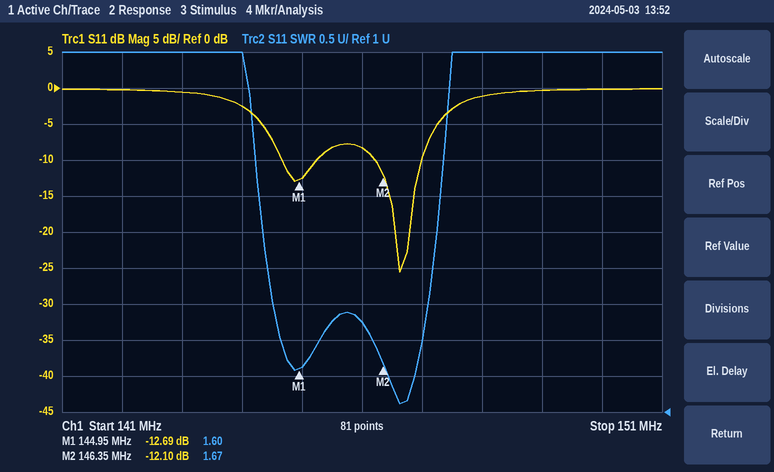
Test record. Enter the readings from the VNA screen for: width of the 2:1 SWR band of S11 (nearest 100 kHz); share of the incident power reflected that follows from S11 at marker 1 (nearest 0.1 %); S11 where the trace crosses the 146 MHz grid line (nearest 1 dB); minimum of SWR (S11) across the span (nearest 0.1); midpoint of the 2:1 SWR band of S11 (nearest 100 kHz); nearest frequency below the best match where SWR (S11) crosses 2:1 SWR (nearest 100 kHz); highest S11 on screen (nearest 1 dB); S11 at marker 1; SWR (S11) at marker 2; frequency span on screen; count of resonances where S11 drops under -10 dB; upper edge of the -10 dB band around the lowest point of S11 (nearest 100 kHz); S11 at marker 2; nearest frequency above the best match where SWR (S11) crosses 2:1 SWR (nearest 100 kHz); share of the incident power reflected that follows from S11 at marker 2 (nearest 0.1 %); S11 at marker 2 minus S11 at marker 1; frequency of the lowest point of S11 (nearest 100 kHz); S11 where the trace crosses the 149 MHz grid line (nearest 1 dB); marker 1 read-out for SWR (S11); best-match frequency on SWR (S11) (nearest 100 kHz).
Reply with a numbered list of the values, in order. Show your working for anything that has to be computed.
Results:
1. 147.0 MHz − 146.2 MHz = 800 kHz
2. 10^(-12.69/10) ≈ 5.4 %
3. -8 dB
4. 1.1
5. 146.6 MHz
6. 146.2 MHz
7. 0 dB
8. -12.69 dB
9. 1.67
10. 10 MHz
11. 2
12. 147.0 MHz
13. -12.10 dB
14. 147.0 MHz
15. 10^(-12.1/10) ≈ 6.2 %
16. -12.1 − (-12.69) = 0.59 dB
17. 146.6 MHz
18. 0 dB
19. 1.60
20. 146.6 MHz
